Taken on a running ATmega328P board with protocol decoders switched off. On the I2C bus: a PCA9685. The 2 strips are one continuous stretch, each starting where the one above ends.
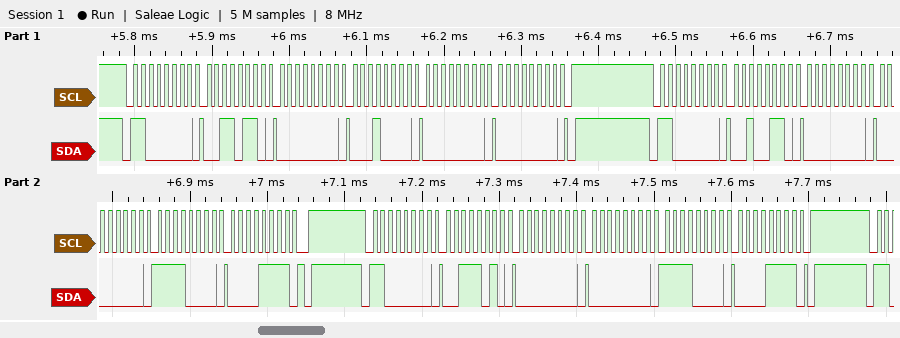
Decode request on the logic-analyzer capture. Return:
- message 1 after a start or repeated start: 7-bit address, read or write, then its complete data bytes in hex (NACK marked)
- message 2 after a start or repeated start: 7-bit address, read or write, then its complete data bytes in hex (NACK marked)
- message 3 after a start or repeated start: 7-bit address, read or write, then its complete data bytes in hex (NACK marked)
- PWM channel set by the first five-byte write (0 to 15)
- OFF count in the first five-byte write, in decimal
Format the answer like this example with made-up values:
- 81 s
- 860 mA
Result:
- 0x60 write: 36 00 10 00 00
- 0x60 write: 26 00 00 F0 0F
- 0x60 write: 3A 00 00 F0 0F
- 12
- 0
